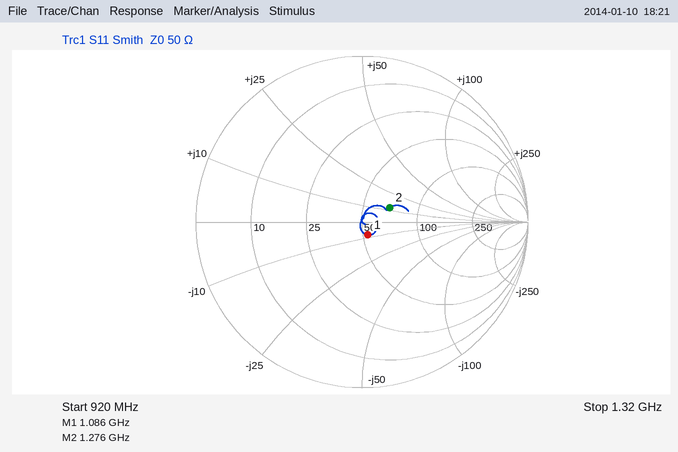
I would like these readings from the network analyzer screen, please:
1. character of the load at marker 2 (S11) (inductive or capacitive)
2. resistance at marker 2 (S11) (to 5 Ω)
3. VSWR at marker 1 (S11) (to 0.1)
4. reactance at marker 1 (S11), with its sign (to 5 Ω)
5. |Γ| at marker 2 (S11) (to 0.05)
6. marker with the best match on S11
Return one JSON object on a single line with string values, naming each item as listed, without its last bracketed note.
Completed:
{"character of the load at marker 2 (S11)": "inductive", "resistance at marker 2 (S11)": "70 Ω", "VSWR at marker 1 (S11)": "1.2", "reactance at marker 1 (S11), with its sign": "-10 Ω", "|Γ| at marker 2 (S11)": "0.20", "marker with the best match on S11": "marker 1"}
